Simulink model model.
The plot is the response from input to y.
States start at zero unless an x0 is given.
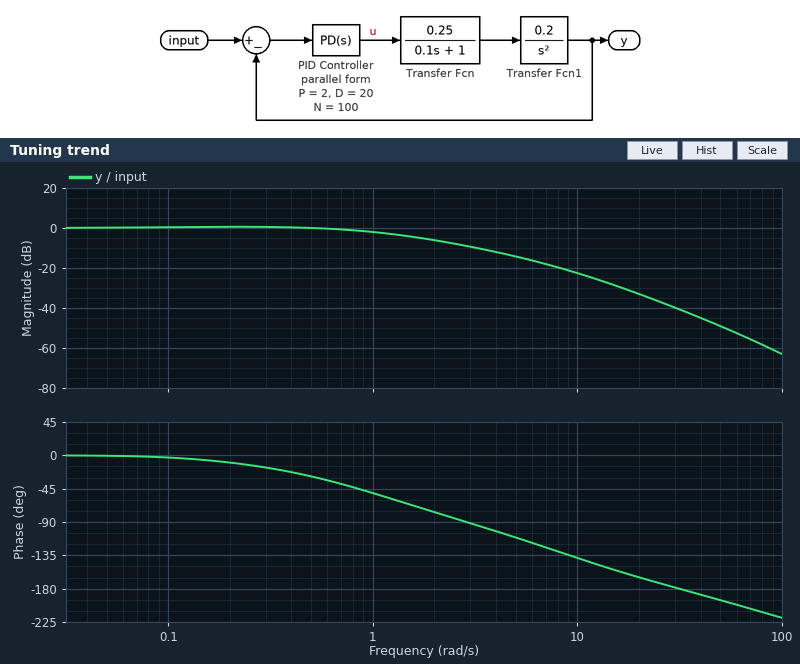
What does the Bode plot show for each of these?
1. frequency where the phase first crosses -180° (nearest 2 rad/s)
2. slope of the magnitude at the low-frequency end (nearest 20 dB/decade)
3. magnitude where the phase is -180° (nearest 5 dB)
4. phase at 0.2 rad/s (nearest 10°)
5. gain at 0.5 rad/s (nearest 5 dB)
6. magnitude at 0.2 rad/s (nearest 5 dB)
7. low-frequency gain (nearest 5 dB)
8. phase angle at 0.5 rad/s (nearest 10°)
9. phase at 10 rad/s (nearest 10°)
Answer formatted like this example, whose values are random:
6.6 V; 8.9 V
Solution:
32 rad/s; 0 dB/decade; -40 dB; -10°; 0 dB; 0 dB; 0 dB; -30°; -140°
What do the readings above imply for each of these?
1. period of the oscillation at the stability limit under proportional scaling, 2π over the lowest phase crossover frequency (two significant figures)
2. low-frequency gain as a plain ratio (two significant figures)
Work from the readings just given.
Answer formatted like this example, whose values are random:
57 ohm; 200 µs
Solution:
0.20 s; 1.0
